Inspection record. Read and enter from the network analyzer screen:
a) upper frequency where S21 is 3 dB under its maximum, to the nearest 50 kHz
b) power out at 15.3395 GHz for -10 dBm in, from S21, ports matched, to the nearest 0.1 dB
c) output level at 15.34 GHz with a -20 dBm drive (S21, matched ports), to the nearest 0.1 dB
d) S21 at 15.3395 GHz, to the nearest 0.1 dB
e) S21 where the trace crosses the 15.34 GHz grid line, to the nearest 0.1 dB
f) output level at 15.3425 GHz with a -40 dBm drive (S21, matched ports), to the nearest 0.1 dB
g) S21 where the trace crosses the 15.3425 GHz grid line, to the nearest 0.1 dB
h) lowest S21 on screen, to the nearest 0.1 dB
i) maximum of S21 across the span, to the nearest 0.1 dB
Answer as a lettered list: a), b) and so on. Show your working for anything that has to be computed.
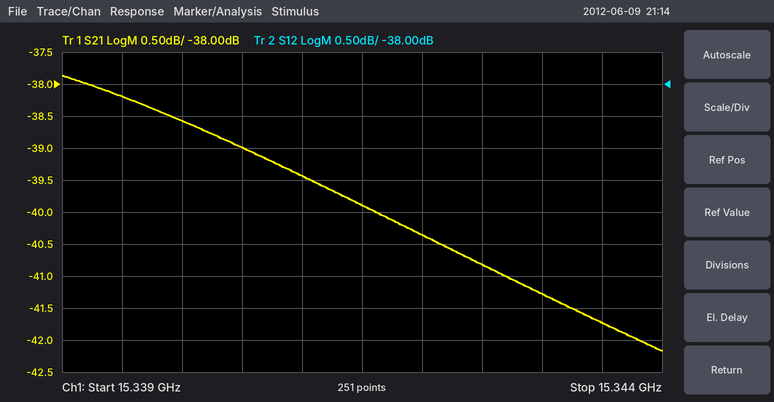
a) 15.34255 GHz
b) -10 dBm + (-38.2 dB) = -48.2 dBm
c) -20 dBm + (-38.6 dB) = -58.6 dBm
d) -38.2 dB
e) -38.6 dB
f) -40 dBm + (-40.8 dB) = -80.8 dBm
g) -40.8 dB
h) -42.2 dB
i) -37.9 dB
